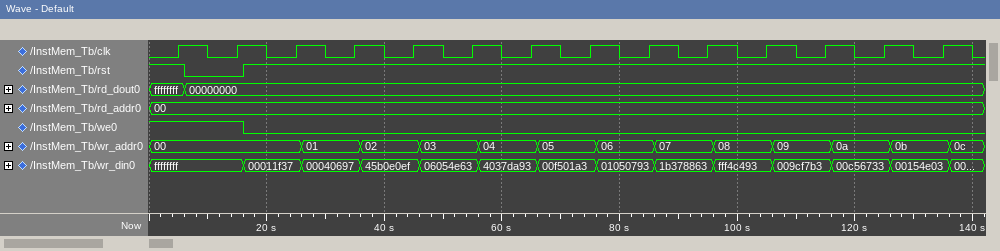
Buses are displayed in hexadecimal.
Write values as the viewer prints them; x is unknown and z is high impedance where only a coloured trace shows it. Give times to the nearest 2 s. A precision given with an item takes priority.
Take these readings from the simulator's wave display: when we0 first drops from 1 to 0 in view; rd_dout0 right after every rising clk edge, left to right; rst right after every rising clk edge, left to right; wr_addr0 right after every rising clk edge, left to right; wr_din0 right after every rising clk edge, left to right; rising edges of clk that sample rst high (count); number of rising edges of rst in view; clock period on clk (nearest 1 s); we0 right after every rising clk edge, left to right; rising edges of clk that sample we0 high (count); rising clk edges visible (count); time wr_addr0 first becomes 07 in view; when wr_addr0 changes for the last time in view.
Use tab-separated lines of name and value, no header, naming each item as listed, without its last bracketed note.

when we0 first drops from 1 to 0 in view	16 s
rd_dout0 right after every rising clk edge, left to right	ffffffff, 00000000, 00000000, 00000000, 00000000, 00000000, 00000000, 00000000, 00000000, 00000000, 00000000, 00000000, 00000000, 00000000
rst right after every rising clk edge, left to right	1 0 1 1 1 1 1 1 1 1 1 1 1 1
wr_addr0 right after every rising clk edge, left to right	00, 00, 00, 01, 02, 03, 04, 05, 06, 07, 08, 09, 0a, 0b
wr_din0 right after every rising clk edge, left to right	ffffffff, ffffffff, 00011f37, 00040697, 45b0e0ef, 06054e63, 4037da93, 00f501a3, 01050793, 1b378863, fff4c493, 009cf7b3, 00c56733, 00154e03
rising edges of clk that sample rst high	13
number of rising edges of rst in view	1
clock period on clk	10 s
we0 right after every rising clk edge, left to right	1 1 0 0 0 0 0 0 0 0 0 0 0 0
rising edges of clk that sample we0 high	2
rising clk edges visible	14
time wr_addr0 first becomes 07 in view	86 s
when wr_addr0 changes for the last time in view	136 s
